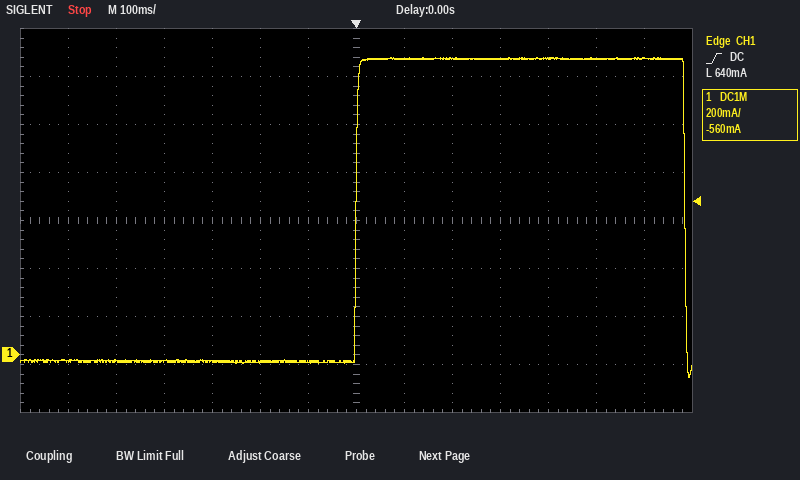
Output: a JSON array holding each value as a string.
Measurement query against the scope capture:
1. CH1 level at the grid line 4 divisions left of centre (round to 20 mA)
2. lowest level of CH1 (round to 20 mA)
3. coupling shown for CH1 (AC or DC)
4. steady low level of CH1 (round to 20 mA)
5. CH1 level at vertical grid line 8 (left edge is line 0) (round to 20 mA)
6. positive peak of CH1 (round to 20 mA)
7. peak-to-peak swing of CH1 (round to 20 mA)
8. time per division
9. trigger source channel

["-20 mA", "-100 mA", "DC", "-20 mA", "1.24 A", "1.24 A", "1.34 A", "100 ms", "CH1"]
